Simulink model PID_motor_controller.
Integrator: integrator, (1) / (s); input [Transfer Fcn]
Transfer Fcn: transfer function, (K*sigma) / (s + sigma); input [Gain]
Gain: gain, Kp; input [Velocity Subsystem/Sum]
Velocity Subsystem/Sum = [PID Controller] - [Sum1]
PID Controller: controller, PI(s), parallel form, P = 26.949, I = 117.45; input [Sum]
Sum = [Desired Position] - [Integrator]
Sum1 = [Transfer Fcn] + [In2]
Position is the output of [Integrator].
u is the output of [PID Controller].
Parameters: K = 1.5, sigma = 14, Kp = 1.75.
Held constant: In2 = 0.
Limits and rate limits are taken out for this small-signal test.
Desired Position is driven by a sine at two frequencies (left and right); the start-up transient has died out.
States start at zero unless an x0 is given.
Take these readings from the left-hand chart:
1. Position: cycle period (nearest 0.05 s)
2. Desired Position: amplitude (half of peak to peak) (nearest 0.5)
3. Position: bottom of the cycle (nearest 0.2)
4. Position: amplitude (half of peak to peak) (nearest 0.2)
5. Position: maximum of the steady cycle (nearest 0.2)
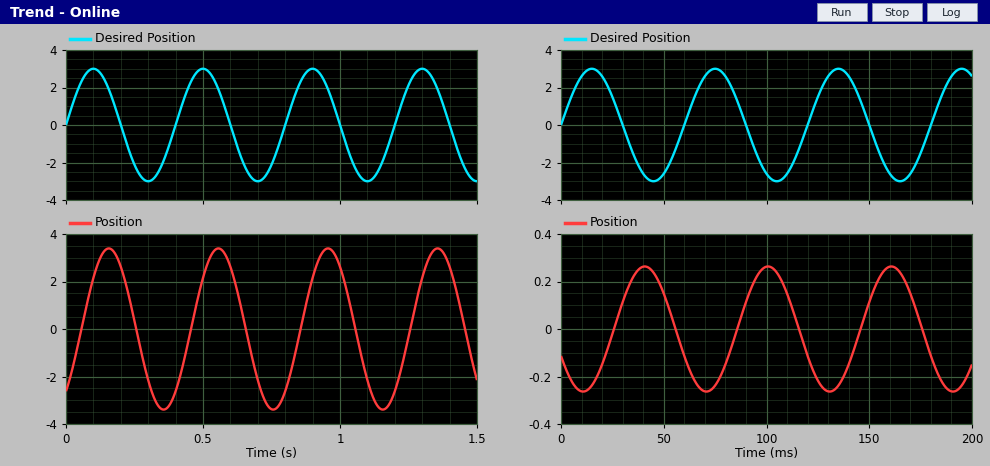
0.40 s
3.0
-3.4
3.4
3.4
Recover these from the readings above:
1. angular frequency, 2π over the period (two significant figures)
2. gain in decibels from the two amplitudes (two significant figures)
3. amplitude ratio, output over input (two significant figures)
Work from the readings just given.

16 rad/s
1.1 dB
1.1
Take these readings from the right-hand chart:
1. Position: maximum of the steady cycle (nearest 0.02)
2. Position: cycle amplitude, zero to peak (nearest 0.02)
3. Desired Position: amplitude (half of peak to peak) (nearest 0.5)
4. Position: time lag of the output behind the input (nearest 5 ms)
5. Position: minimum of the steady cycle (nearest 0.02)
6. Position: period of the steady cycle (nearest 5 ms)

0.26
0.26
3.0
25 ms
-0.26
60 ms
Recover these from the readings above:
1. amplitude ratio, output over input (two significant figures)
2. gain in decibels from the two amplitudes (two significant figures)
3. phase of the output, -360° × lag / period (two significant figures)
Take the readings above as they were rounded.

0.087
-21 dB
-150°
